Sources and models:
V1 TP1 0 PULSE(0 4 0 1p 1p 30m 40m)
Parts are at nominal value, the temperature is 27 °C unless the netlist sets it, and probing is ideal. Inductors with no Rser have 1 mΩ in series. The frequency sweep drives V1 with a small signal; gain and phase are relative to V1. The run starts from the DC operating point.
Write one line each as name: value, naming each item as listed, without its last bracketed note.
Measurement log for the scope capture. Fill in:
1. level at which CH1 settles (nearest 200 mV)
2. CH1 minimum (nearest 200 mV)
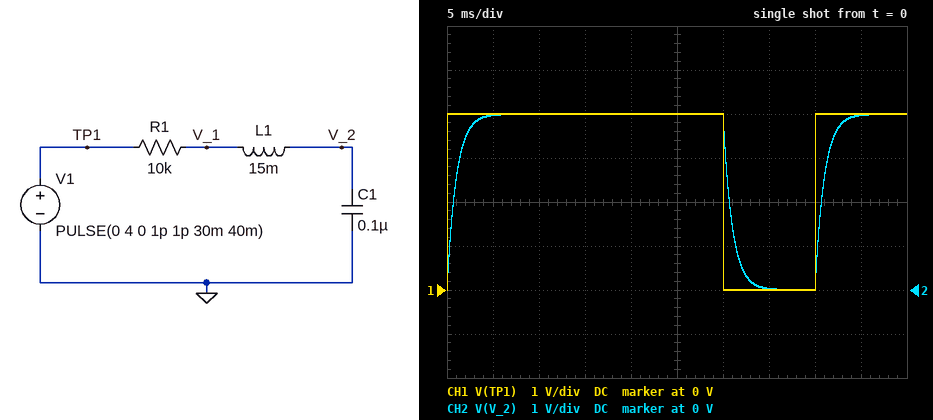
level at which CH1 settles: 4.0 V
CH1 minimum: 0 V
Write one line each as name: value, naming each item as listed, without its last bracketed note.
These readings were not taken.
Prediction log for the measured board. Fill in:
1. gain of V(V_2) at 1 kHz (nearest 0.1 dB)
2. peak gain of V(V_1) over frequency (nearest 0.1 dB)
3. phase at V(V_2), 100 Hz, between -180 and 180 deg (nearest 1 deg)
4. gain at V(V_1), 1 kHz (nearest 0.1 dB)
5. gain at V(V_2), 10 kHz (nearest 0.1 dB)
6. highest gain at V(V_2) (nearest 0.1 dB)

gain of V(V_2) at 1 kHz: -16.1 dB
peak gain of V(V_1) over frequency: 0 dB
phase at V(V_2), 100 Hz, between -180 and 180 deg: -32 deg
gain at V(V_1), 1 kHz: -16.6 dB
gain at V(V_2), 10 kHz: -36.0 dB
highest gain at V(V_2): 0 dB
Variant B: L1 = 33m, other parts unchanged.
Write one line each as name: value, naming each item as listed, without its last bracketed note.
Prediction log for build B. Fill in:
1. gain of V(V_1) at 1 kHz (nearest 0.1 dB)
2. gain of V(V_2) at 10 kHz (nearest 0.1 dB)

gain of V(V_1) at 1 kHz: -17.3 dB
gain of V(V_2) at 10 kHz: -36.1 dB
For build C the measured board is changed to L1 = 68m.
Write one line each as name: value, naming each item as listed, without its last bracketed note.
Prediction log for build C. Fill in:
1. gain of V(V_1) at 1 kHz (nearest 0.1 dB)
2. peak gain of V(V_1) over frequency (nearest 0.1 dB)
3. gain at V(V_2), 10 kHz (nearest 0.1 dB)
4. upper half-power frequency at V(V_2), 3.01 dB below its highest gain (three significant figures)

gain of V(V_1) at 1 kHz: -18.7 dB
peak gain of V(V_1) over frequency: 0 dB
gain at V(V_2), 10 kHz: -36.6 dB
upper half-power frequency at V(V_2), 3.01 dB below its highest gain: 160 Hz
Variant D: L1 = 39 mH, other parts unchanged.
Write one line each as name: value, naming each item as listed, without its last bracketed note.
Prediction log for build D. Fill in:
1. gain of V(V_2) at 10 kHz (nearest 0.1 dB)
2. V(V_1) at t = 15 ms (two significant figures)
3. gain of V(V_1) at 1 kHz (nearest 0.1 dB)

gain of V(V_2) at 10 kHz: -36.2 dB
V(V_1) at t = 15 ms: 4.0 V
gain of V(V_1) at 1 kHz: -17.5 dB
